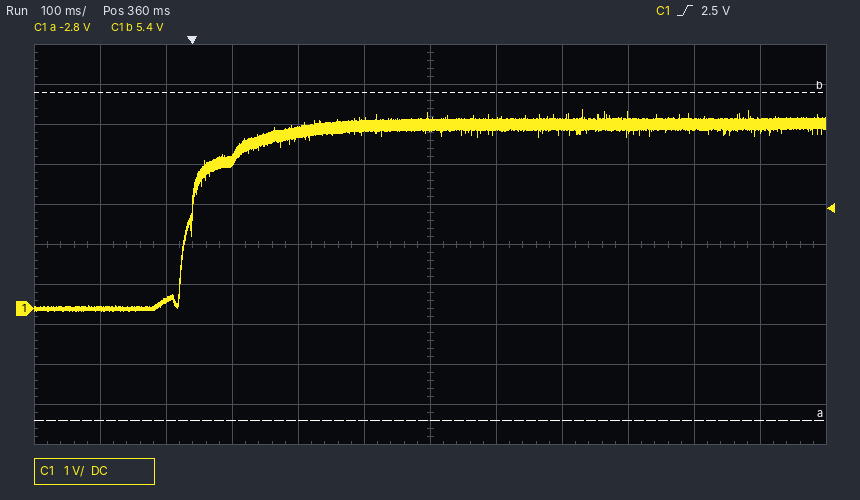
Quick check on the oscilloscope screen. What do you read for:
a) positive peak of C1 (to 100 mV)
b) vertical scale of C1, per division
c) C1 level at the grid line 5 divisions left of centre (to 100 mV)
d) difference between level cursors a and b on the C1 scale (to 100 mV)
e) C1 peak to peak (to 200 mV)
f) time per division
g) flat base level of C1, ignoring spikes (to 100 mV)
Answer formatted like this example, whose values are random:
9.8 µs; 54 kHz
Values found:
5.0 V; 1 V; 0.0 V; 8.2 V; 5.0 V; 100 ms; 0.0 V
